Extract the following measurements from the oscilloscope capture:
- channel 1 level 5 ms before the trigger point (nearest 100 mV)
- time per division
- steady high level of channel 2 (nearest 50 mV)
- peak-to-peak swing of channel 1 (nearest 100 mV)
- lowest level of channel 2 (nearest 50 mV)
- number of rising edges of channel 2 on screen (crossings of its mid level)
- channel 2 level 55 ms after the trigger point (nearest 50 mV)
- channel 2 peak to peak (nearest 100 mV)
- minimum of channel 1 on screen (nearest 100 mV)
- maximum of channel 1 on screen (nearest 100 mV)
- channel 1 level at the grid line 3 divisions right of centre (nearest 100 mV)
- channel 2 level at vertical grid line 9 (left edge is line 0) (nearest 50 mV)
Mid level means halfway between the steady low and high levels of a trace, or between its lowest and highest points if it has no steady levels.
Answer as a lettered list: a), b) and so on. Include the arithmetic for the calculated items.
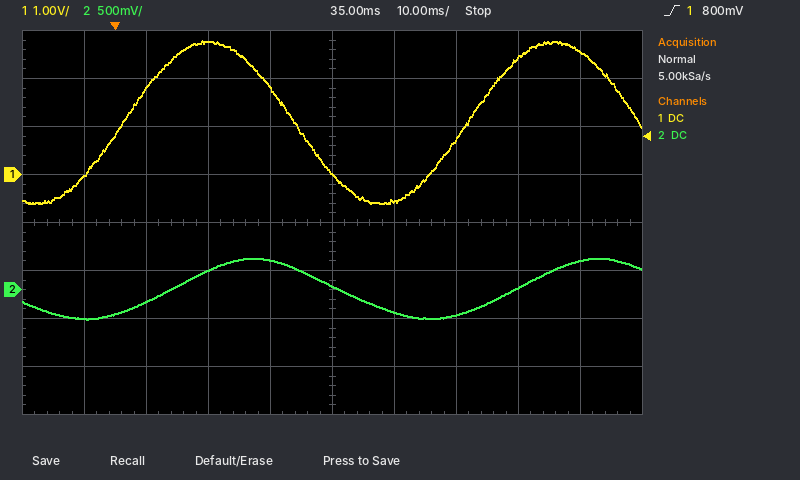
a) 0.0 V
b) 10 ms
c) 300 mV
d) 2.8 V − (-600 mV) = 3.4 V
e) -300 mV
f) 2
g) -250 mV
h) 600 mV
i) -600 mV
j) 2.8 V
k) 2.4 V
l) 300 mV
